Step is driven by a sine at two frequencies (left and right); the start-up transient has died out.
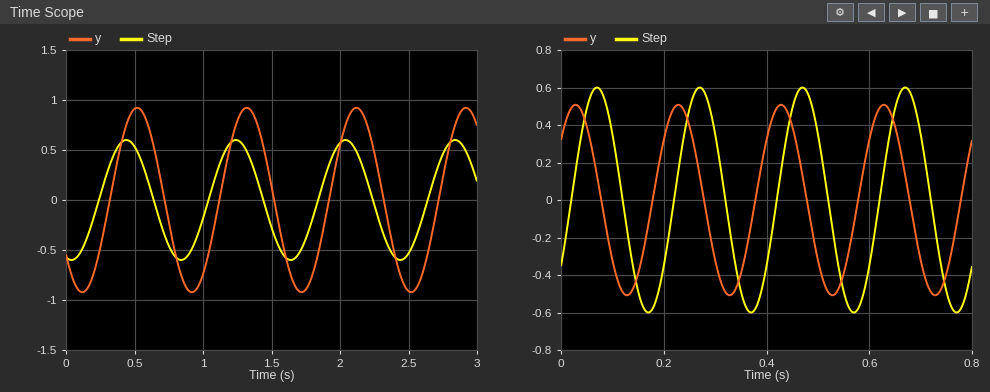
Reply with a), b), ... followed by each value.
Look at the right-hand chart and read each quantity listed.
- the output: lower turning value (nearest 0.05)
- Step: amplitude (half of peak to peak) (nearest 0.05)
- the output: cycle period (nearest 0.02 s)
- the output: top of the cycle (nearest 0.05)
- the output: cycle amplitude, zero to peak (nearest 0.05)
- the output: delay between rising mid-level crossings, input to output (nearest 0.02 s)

a) -0.50
b) 0.60
c) 0.20 s
d) 0.50
e) 0.50
f) 0.16 s
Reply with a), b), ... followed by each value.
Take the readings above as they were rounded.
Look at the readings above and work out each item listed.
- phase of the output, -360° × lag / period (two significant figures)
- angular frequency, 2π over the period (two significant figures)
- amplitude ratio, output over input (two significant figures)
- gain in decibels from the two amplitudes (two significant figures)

a) -290°
b) 31 rad/s
c) 0.83
d) -1.6 dB
